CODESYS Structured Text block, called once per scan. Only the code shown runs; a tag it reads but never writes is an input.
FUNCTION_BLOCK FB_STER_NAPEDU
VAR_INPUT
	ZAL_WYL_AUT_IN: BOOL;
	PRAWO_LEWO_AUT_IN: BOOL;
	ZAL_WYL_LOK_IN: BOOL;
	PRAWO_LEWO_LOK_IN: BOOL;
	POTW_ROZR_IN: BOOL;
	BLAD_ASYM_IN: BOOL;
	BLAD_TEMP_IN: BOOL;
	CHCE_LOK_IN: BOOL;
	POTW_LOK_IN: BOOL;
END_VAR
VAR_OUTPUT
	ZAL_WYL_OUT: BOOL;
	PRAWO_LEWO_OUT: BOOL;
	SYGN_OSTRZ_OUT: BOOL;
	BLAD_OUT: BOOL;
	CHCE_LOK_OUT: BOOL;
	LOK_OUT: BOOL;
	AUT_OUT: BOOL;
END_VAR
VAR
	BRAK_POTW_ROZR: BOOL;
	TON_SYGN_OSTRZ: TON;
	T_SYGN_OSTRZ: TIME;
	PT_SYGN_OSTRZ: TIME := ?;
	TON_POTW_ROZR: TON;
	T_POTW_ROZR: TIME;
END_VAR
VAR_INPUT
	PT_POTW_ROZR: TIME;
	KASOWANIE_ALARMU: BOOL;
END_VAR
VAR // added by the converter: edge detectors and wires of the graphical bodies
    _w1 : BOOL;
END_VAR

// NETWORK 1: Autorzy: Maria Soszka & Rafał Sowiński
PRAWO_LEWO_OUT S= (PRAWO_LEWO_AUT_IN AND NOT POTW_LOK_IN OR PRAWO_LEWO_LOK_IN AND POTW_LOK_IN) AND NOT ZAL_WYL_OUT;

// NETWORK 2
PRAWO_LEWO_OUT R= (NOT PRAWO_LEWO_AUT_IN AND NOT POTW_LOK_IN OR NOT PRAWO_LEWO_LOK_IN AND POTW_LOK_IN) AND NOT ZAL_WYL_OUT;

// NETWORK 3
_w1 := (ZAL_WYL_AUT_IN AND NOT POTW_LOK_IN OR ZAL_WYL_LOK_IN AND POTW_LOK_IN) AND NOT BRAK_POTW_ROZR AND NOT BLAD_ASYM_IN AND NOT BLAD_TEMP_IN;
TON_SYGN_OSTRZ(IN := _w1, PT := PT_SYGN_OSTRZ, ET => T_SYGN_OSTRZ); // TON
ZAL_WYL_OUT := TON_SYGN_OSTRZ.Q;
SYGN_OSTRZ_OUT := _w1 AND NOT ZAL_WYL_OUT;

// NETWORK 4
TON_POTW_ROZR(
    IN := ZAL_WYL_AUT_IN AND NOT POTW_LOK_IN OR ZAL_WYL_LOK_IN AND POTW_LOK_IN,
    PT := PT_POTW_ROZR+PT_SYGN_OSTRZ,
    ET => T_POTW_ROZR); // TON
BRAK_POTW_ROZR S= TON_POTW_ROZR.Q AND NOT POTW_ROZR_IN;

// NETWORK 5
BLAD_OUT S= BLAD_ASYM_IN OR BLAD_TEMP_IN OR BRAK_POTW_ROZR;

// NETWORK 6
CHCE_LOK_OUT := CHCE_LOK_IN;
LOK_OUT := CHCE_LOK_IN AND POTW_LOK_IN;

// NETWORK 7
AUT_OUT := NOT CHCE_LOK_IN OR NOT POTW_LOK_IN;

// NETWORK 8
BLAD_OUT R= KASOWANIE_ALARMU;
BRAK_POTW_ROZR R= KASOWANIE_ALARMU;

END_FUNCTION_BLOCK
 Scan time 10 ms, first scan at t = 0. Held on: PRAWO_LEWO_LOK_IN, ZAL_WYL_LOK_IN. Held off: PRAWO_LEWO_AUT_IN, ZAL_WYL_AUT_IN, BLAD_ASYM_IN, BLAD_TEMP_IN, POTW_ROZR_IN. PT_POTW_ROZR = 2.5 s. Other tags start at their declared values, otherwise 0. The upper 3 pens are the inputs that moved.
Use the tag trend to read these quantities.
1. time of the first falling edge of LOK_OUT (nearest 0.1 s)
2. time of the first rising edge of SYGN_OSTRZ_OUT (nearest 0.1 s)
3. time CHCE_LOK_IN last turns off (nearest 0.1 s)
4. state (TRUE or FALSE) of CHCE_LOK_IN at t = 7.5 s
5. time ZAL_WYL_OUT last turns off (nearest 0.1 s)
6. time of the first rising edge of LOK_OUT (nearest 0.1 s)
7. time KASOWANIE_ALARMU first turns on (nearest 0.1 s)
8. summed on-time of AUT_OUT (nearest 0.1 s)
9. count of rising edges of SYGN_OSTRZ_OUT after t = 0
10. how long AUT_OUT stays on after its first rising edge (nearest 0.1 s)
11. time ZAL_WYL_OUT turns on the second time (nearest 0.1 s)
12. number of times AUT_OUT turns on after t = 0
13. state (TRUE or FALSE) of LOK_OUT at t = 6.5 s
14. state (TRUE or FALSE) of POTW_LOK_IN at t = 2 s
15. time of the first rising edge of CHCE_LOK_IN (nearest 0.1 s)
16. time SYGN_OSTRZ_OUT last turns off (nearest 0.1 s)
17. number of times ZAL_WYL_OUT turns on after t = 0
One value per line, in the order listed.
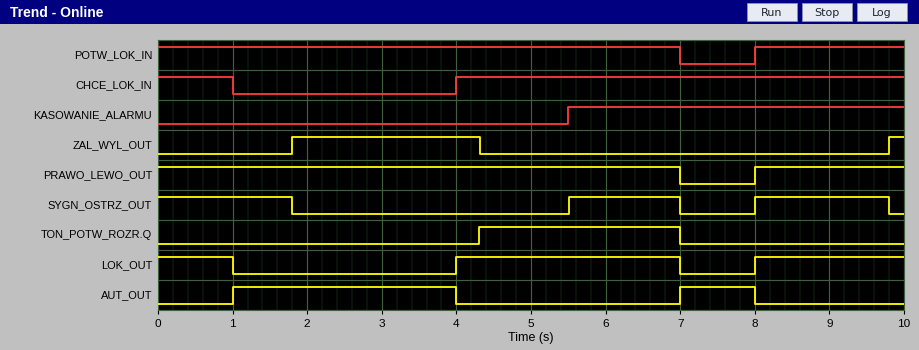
1.0 s
5.5 s
1.0 s
TRUE
4.3 s
4.0 s
5.5 s
4.0 s
2
3.0 s
9.8 s
2
TRUE
TRUE
4.0 s
9.8 s
2
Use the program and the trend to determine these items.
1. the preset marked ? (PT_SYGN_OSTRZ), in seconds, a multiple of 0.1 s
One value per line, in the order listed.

1.8 s
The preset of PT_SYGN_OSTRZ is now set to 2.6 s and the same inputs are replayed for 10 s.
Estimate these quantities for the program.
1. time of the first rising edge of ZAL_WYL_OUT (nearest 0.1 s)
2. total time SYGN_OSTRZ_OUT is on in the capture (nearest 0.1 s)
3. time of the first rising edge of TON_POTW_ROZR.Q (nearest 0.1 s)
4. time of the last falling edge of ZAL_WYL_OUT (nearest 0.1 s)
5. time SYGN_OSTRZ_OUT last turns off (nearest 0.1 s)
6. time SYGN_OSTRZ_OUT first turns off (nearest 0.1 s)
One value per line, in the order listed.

2.6 s
6.1 s
5.1 s
5.1 s
7.0 s
2.6 s
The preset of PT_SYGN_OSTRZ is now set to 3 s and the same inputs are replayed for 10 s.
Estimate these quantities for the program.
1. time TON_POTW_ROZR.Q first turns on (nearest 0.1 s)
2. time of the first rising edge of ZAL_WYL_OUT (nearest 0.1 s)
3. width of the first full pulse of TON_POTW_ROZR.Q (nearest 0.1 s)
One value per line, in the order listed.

5.5 s
3.0 s
1.5 s
